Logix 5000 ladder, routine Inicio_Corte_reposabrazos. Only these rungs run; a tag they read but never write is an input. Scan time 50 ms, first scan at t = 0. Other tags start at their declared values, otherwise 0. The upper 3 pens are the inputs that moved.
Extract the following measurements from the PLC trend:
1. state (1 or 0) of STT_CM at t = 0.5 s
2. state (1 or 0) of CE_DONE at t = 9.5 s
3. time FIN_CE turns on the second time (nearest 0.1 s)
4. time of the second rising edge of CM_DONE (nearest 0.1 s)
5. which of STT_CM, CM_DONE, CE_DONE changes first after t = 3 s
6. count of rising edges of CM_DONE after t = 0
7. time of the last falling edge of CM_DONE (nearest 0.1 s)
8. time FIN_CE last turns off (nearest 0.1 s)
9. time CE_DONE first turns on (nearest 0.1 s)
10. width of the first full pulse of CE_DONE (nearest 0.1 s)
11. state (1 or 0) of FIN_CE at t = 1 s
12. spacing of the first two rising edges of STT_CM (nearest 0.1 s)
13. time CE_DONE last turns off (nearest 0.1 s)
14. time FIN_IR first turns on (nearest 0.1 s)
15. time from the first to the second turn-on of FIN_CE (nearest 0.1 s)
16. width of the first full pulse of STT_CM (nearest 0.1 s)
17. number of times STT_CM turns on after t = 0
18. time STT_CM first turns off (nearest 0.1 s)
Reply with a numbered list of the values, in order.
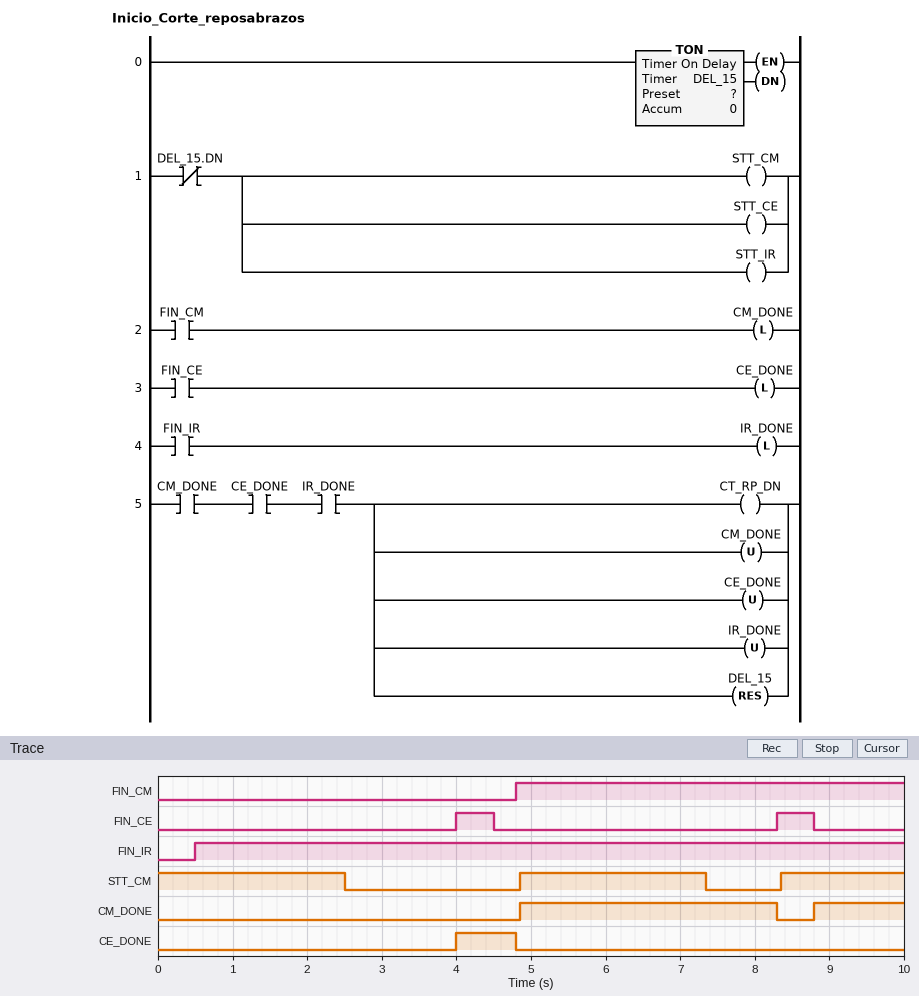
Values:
1. 1
2. 0
3. 8.3 s
4. 8.8 s
5. CE_DONE
6. 2
7. 8.3 s
8. 8.8 s
9. 4.0 s
10. 0.8 s
11. 0
12. 3.5 s
13. 4.8 s
14. 0.5 s
15. 4.3 s
16. 2.5 s
17. 2
18. 2.5 s
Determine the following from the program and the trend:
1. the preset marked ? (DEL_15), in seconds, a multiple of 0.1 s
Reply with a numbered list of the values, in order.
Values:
1. 2.5 s
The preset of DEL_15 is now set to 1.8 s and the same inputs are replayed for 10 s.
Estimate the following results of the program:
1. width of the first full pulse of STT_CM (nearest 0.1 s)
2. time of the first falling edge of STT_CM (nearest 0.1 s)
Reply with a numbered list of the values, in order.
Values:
1. 1.8 s
2. 1.8 s
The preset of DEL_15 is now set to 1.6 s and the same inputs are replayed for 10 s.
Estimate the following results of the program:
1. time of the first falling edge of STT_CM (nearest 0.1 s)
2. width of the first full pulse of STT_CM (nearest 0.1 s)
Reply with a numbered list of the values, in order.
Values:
1. 1.6 s
2. 1.6 s
